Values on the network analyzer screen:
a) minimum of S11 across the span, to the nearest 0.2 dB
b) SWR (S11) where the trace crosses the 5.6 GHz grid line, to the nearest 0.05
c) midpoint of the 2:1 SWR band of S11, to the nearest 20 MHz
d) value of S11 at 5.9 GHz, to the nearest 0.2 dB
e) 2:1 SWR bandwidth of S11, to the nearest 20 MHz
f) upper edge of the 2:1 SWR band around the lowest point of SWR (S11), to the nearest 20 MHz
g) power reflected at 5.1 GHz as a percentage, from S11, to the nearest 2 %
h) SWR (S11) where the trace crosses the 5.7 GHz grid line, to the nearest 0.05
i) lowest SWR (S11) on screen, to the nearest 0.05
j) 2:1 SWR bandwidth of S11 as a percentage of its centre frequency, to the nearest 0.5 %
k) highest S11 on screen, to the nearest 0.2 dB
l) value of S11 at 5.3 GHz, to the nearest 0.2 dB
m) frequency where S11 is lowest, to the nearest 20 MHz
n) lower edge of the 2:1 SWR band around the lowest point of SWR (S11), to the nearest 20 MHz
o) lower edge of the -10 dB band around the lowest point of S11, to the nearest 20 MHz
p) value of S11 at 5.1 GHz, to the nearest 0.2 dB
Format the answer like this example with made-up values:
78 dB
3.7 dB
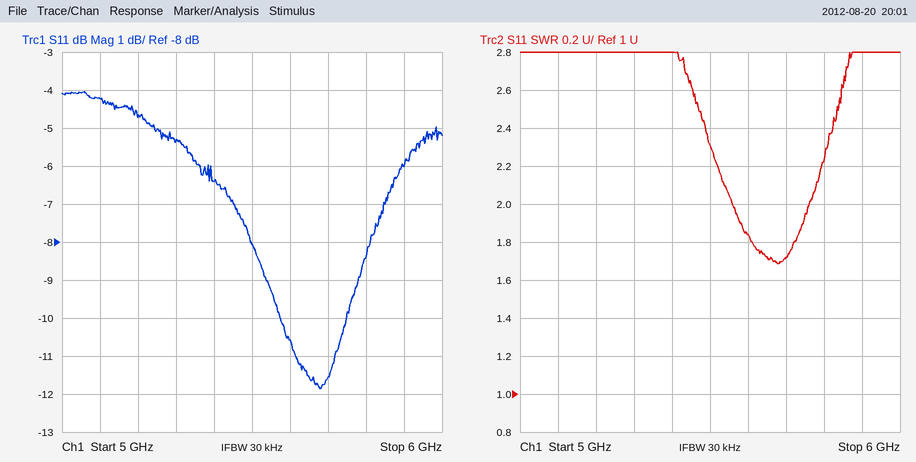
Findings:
-11.8 dB
1.85
5.66 GHz
-6.0 dB
200 MHz
5.76 GHz
38 %
1.70
1.70
3.5 %
-4.0 dB
-5.4 dB
5.68 GHz
5.56 GHz
5.58 GHz
-4.2 dB
